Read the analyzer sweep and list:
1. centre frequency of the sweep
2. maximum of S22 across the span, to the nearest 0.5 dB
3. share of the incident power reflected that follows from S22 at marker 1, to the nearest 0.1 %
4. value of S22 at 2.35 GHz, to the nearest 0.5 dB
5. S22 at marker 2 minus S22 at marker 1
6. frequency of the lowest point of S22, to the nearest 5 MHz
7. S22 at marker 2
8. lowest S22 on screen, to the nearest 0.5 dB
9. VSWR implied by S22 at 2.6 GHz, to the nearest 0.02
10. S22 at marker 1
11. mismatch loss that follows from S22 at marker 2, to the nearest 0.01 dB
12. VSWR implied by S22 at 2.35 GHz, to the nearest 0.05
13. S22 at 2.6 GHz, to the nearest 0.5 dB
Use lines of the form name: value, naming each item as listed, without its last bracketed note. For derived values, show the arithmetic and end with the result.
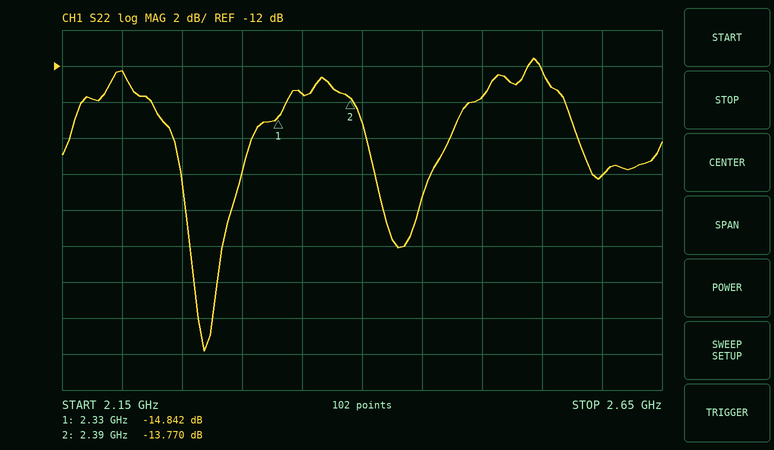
centre frequency of the sweep: 2.4 GHz
maximum of S22 across the span, to the nearest 0.5 dB: -11.5 dB
share of the incident power reflected that follows from S22 at marker 1, to the nearest 0.1 %: 10^(-14.842/10) ≈ 3.3 %
value of S22 at 2.35 GHz, to the nearest 0.5 dB: -13.5 dB
S22 at marker 2 minus S22 at marker 1: -13.77 − (-14.842) = 1.072 dB
frequency of the lowest point of S22, to the nearest 5 MHz: 2.270 GHz
S22 at marker 2: -13.770 dB
lowest S22 on screen, to the nearest 0.5 dB: -28.0 dB
VSWR implied by S22 at 2.6 GHz, to the nearest 0.02: |Γ| = 10^(-18/20) = 0.1259; VSWR = (1 + 0.1259)/(1 − 0.1259) ≈ 1.29, so 1.28 to the nearest 0.02
S22 at marker 1: -14.842 dB
mismatch loss that follows from S22 at marker 2, to the nearest 0.01 dB: −10 log10(1 − 10^(-13.77/10)) ≈ 0.19 dB
VSWR implied by S22 at 2.35 GHz, to the nearest 0.05: |Γ| = 10^(-13.5/20) = 0.2113; VSWR = (1 + 0.2113)/(1 − 0.2113) ≈ 1.54, so 1.55 to the nearest 0.05
S22 at 2.6 GHz, to the nearest 0.5 dB: -18.0 dB
